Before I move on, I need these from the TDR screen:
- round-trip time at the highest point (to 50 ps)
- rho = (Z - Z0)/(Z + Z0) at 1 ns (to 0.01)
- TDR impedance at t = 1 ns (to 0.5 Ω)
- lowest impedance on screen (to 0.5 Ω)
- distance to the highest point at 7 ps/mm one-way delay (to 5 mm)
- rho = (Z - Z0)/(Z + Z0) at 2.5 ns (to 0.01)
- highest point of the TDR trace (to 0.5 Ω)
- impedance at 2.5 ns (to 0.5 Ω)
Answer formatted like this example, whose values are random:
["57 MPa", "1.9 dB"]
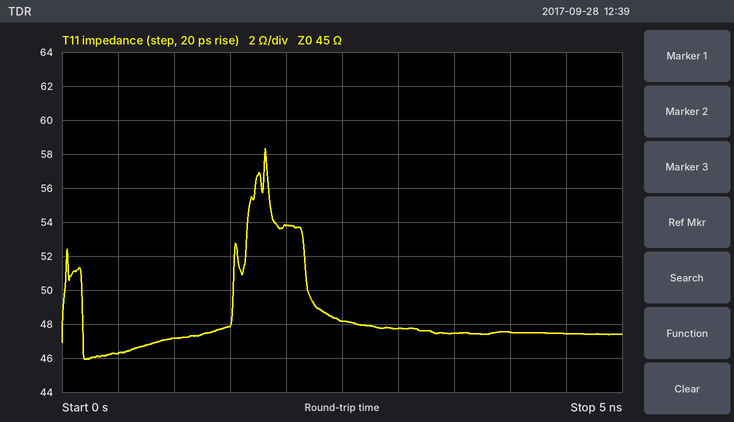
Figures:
["1.80 ns", "+0.02", "47.0 Ω", "46.0 Ω", "130 mm", "+0.03", "58.5 Ω", "48.0 Ω"]
